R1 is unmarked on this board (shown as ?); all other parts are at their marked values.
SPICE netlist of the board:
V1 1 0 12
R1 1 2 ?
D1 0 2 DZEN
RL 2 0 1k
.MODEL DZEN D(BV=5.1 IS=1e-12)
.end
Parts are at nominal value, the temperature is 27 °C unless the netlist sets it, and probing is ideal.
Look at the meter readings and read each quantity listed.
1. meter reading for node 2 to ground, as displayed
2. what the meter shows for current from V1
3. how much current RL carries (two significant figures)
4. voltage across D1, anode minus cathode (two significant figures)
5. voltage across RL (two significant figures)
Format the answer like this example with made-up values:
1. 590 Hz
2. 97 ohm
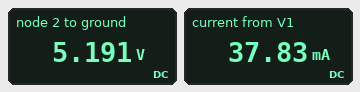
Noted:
1. 5.191 V
2. 37.83 mA
3. 5.2 mA
4. -5.2 V
5. 5.2 V
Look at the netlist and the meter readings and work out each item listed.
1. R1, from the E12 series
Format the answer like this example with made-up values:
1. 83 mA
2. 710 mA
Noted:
1. 180 Ω
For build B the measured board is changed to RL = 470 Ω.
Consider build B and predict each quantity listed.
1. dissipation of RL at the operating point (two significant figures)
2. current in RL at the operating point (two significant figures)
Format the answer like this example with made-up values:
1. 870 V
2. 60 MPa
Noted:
1. 57 mW
2. 11 mA
